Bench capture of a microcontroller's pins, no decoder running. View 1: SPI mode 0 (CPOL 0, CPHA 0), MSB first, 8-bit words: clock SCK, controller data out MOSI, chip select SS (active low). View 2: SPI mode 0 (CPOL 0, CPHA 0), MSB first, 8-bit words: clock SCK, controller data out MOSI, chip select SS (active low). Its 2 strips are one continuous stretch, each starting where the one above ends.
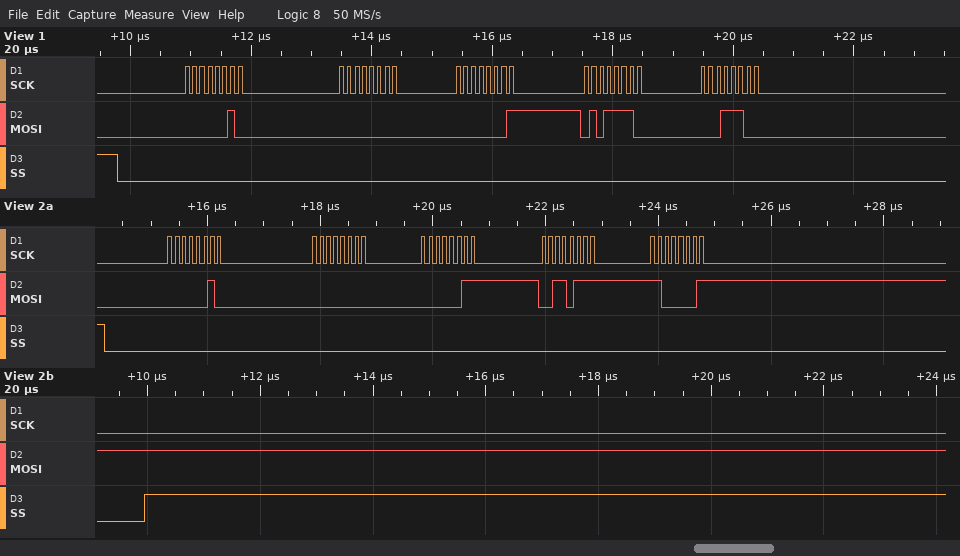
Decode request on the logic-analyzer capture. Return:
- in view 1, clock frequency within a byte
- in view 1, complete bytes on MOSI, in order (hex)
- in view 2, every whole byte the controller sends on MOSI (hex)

8 MHz
02 00 01 5E 1C
02 00 03 37 C1
